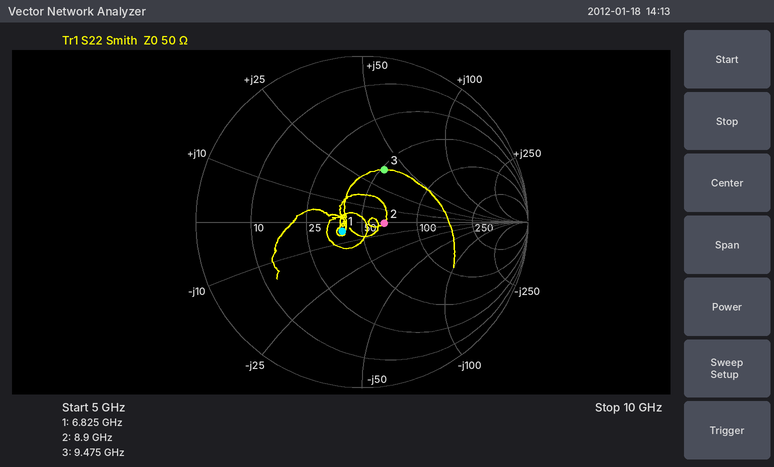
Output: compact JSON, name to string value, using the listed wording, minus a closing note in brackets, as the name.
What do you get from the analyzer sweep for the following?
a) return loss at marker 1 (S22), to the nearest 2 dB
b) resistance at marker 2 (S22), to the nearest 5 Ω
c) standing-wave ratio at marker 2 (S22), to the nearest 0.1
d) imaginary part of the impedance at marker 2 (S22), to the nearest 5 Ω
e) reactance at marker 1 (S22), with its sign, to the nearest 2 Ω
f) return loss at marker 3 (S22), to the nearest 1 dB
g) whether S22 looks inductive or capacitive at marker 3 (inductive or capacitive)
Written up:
{"return loss at marker 1 (S22), to the nearest 2 dB": "18 dB", "resistance at marker 2 (S22), to the nearest 5 Ω": "65 Ω", "standing-wave ratio at marker 2 (S22), to the nearest 0.1": "1.3", "imaginary part of the impedance at marker 2 (S22), to the nearest 5 Ω": "0 Ω", "reactance at marker 1 (S22), with its sign, to the nearest 2 Ω": "-4 Ω", "return loss at marker 3 (S22), to the nearest 1 dB": "9 dB", "whether S22 looks inductive or capacitive at marker 3": "inductive"}
